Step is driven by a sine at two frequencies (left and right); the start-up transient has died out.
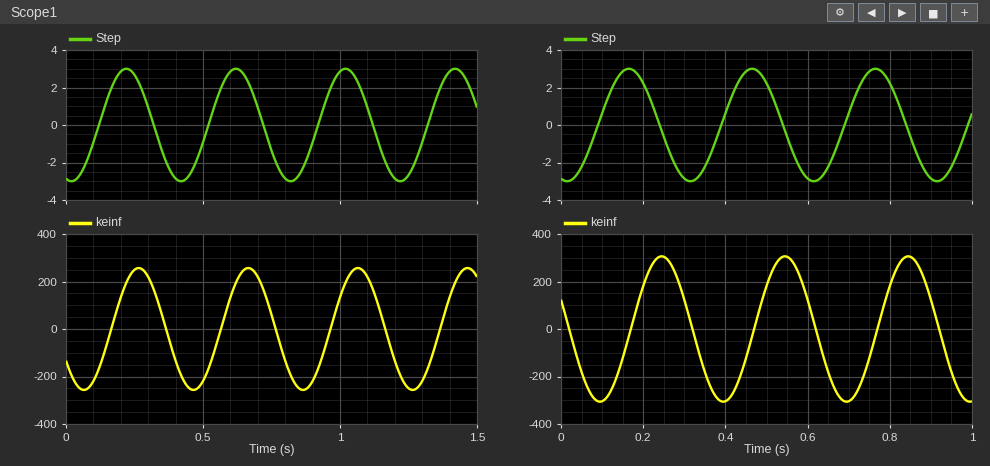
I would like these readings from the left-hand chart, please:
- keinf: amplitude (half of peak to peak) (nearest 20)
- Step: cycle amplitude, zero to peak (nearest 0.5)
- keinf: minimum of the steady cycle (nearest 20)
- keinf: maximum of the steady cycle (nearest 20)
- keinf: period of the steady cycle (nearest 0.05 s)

260
3.0
-260
260
0.40 s
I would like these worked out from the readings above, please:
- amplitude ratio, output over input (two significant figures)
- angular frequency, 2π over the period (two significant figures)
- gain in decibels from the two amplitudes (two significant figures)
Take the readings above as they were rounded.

87
16 rad/s
39 dB
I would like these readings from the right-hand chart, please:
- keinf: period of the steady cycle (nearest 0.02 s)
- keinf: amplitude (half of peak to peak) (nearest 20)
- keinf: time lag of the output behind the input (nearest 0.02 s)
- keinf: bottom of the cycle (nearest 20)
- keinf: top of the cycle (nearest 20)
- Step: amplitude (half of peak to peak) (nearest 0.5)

0.30 s
300
0.08 s
-300
300
3.0
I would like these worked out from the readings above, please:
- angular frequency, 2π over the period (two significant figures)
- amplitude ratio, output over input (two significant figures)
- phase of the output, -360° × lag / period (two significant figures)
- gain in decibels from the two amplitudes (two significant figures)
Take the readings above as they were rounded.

21 rad/s
100
-96°
40 dB
